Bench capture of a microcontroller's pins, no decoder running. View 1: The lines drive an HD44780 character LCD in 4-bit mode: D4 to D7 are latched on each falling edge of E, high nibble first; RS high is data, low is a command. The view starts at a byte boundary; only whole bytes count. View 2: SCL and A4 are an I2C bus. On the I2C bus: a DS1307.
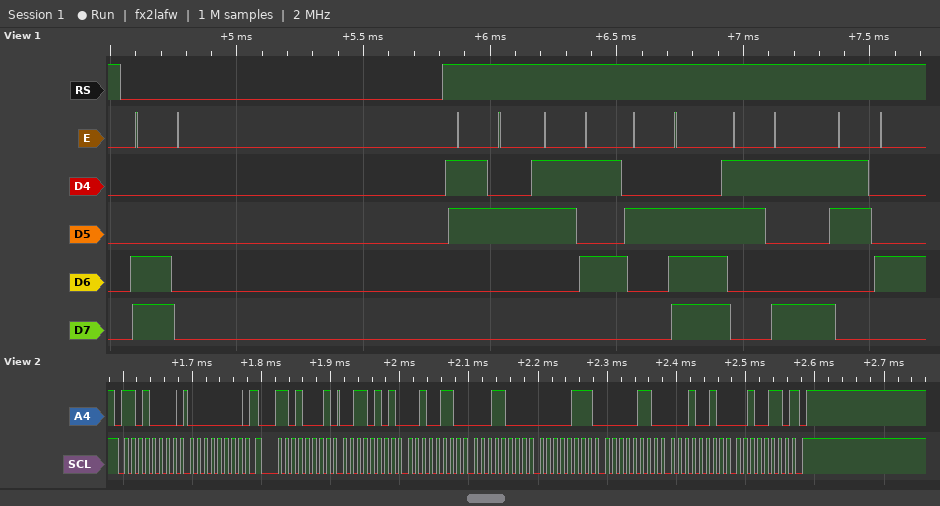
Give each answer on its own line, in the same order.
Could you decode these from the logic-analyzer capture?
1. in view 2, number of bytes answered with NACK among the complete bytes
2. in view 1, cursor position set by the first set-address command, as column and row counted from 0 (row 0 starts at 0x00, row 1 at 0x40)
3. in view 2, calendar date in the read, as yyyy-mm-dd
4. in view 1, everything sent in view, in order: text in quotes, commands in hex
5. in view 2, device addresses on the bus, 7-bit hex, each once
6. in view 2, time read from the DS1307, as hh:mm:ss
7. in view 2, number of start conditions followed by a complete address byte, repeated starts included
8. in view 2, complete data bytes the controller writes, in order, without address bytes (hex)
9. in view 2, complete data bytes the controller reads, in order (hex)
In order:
1
column 0, row 1
2026-12-06
0xC0 "25.94"
0x68
18:26:35
2
00
35 26 18 07 06 12 26
